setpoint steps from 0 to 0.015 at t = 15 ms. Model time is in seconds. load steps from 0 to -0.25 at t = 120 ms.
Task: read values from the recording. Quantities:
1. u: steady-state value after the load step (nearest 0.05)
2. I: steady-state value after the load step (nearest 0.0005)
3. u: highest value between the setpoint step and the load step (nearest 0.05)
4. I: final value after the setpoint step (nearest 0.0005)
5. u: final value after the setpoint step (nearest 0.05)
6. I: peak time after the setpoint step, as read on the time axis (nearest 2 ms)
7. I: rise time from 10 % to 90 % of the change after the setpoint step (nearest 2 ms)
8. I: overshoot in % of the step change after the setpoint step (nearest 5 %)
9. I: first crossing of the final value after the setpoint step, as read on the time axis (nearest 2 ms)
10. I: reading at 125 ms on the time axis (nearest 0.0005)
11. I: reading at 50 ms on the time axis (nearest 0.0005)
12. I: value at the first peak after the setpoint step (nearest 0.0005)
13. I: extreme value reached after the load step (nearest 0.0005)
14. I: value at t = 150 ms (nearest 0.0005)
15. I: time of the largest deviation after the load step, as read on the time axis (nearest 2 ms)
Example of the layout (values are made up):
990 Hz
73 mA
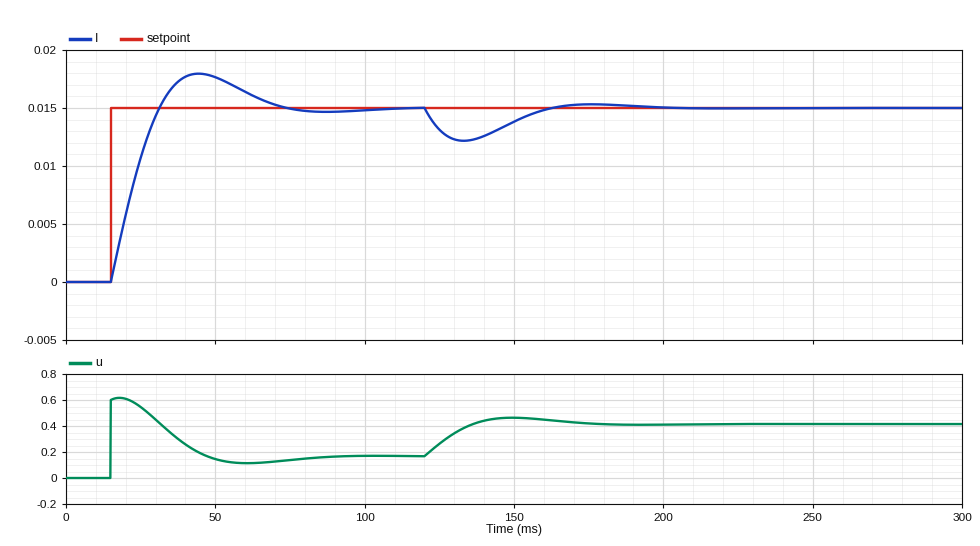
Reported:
0.40
0.0150
0.60
0.0150
0.15
44 ms
12 ms
20 %
32 ms
0.0130
0.0175
0.0180
0.0120
0.0140
134 ms
